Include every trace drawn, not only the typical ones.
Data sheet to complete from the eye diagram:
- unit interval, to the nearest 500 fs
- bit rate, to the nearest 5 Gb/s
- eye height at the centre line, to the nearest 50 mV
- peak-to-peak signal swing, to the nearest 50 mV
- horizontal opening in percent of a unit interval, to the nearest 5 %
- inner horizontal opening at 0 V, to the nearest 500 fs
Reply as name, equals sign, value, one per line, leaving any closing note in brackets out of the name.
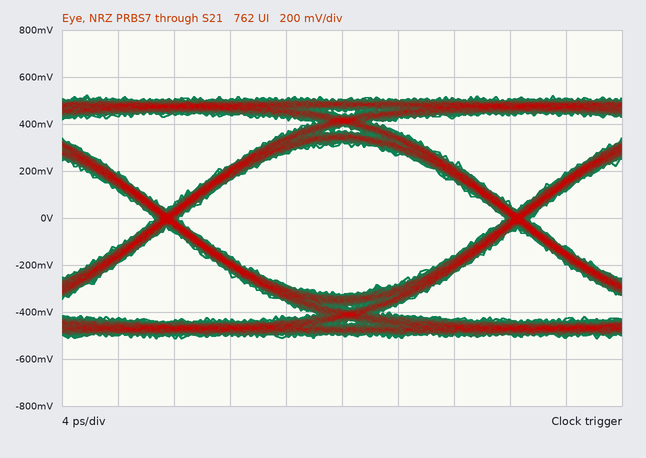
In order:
unit interval, to the nearest 500 fs = 25.0 ps
bit rate, to the nearest 5 Gb/s = 40 Gb/s
eye height at the centre line, to the nearest 50 mV = 650 mV
peak-to-peak signal swing, to the nearest 50 mV = 1.05 V
horizontal opening in percent of a unit interval, to the nearest 5 % = 95 %
inner horizontal opening at 0 V, to the nearest 500 fs = 23.5 ps
